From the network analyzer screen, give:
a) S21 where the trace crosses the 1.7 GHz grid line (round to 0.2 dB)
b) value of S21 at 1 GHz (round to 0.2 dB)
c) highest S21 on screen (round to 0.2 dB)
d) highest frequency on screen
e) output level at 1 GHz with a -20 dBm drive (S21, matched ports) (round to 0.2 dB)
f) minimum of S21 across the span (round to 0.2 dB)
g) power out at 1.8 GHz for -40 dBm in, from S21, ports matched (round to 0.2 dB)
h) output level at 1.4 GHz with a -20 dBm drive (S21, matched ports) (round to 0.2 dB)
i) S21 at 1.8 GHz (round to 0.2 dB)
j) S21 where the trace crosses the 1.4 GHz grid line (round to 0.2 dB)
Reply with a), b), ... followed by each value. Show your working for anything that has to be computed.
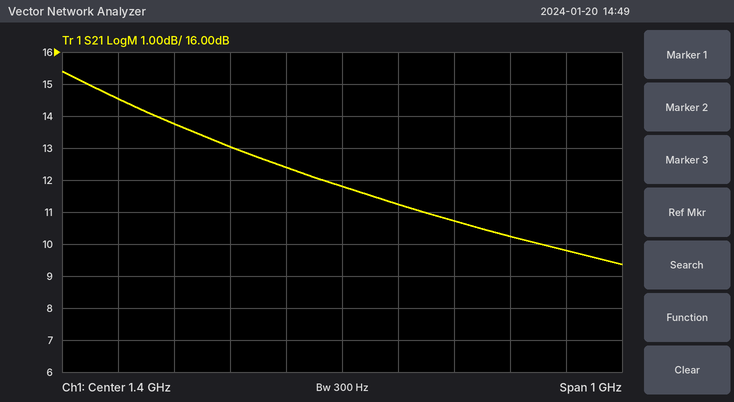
a) 10.2 dB
b) 14.6 dB
c) 15.4 dB
d) 1.9 GHz
e) -20 dBm + (14.6 dB) = -5.4 dBm
f) 9.4 dB
g) -40 dBm + (9.8 dB) = -30.2 dBm
h) -20 dBm + (11.8 dB) = -8.2 dBm
i) 9.8 dB
j) 11.8 dB
